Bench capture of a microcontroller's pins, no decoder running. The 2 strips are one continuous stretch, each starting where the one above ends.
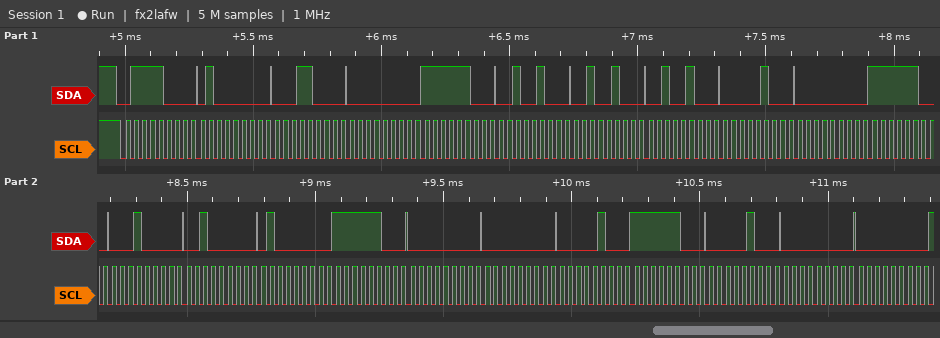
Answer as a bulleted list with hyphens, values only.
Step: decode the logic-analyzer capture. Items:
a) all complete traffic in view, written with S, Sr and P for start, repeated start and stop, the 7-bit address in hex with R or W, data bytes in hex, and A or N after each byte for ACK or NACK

- S 3CW A 40 A 18 A 00 A FC A 24 A 24 A 24 A 04 A 00 A FC A 10 A 20 A 40 A FC A 00 A 00 A 04 A FC A 04 A 00 A 00 A
